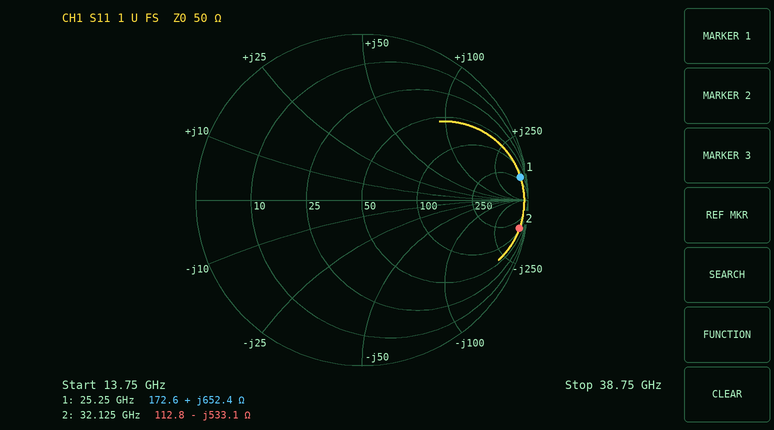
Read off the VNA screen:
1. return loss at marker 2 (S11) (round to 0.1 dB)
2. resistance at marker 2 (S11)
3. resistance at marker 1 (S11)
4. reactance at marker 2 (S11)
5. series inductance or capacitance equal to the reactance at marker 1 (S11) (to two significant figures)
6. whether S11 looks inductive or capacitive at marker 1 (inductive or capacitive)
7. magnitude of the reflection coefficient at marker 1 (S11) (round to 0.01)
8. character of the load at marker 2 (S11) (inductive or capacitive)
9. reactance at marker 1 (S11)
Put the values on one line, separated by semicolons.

0.3 dB; 112.8 Ω; 172.6 Ω; -533.1 Ω; 4.1 nH; inductive; 0.96; capacitive; +652.4 Ω
